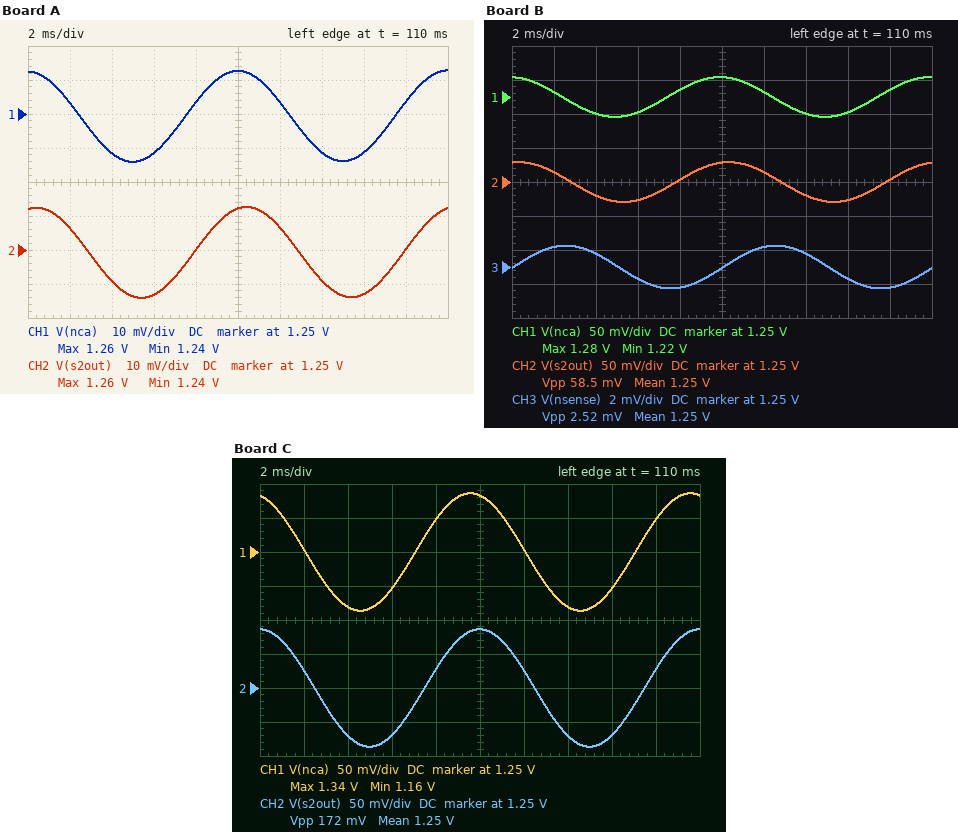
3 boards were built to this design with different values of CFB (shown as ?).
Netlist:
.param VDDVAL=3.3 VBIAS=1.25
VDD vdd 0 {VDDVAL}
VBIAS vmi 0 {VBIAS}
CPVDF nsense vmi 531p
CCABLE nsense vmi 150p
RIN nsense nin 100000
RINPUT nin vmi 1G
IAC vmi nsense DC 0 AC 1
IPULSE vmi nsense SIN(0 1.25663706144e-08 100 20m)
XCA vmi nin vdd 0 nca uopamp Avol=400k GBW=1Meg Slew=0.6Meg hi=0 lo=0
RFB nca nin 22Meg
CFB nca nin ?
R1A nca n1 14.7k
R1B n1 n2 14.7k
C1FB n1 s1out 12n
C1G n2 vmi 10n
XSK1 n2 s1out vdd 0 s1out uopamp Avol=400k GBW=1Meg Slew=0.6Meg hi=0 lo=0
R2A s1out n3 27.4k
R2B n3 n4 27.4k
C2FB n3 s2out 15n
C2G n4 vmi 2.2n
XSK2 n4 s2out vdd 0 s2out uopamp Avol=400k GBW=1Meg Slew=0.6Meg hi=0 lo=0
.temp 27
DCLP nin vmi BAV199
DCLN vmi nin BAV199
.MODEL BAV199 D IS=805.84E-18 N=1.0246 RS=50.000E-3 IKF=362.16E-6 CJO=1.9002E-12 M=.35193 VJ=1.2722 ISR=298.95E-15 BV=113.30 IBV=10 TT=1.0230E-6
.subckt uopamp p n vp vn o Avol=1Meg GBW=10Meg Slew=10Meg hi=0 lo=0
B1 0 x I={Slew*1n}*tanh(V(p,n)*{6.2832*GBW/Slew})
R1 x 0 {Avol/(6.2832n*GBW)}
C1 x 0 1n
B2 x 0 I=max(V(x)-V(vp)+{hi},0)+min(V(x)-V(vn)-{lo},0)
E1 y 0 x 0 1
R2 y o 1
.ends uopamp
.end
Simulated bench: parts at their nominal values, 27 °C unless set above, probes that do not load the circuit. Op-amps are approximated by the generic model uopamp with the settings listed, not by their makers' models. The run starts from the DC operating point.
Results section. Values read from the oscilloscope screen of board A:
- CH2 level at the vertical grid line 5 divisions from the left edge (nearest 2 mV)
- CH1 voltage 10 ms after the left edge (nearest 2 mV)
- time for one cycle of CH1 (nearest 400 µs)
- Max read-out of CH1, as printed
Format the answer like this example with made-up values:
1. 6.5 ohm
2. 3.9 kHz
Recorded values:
1. 1.262 V
2. 1.262 V
3. 10.0 ms
4. 1.26 V
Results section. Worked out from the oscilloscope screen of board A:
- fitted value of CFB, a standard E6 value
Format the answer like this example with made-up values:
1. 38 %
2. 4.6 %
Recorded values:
1. 1.5 nF
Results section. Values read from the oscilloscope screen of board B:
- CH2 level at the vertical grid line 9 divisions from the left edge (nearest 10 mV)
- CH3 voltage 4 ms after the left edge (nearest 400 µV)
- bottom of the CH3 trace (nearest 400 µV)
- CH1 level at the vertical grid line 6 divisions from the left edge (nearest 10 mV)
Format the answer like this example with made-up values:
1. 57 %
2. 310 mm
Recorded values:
1. 1.25 V
2. 1.2508 V
3. 1.2488 V
4. 1.26 V
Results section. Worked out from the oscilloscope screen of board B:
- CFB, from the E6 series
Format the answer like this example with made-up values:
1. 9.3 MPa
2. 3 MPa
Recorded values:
1. 680 pF
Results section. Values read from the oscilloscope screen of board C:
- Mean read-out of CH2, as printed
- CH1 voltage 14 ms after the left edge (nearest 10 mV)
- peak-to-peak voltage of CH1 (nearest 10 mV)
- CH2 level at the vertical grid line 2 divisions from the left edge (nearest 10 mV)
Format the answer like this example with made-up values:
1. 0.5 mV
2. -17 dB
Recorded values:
1. 1.25 V
2. 1.17 V
3. 170 mV
4. 1.18 V
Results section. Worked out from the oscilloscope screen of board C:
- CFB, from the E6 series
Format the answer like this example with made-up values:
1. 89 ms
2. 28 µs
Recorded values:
1. 220 pF
